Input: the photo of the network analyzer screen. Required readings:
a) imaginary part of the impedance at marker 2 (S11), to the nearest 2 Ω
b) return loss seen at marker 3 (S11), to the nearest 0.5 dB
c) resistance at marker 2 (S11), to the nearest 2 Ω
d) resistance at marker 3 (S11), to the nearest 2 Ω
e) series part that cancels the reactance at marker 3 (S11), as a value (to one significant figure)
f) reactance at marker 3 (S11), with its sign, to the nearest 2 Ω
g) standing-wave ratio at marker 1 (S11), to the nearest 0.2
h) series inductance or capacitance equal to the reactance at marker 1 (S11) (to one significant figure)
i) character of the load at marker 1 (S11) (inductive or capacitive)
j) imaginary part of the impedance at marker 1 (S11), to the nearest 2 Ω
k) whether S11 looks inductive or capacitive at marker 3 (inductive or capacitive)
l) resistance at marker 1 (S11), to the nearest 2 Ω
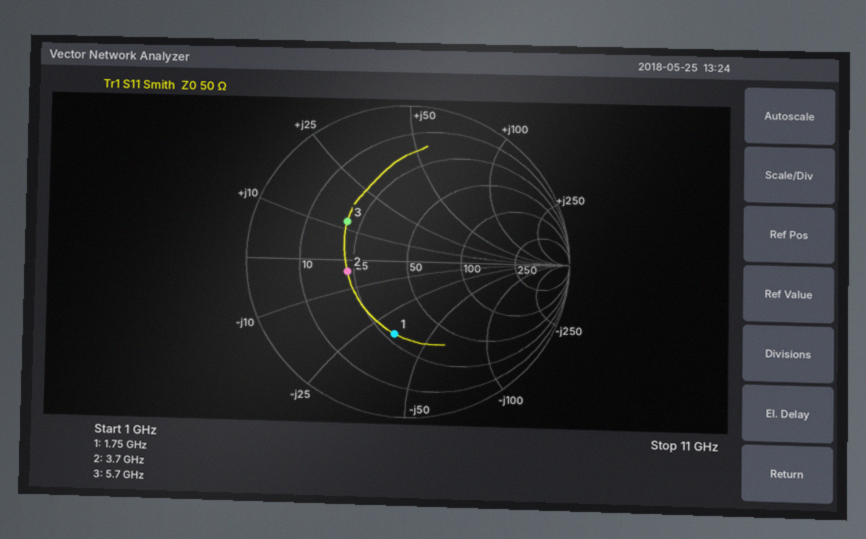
-4 Ω
7.0 dB
22 Ω
20 Ω
2 pF
+12 Ω
2.8
3 pF
capacitive
-34 Ω
inductive
28 Ω
